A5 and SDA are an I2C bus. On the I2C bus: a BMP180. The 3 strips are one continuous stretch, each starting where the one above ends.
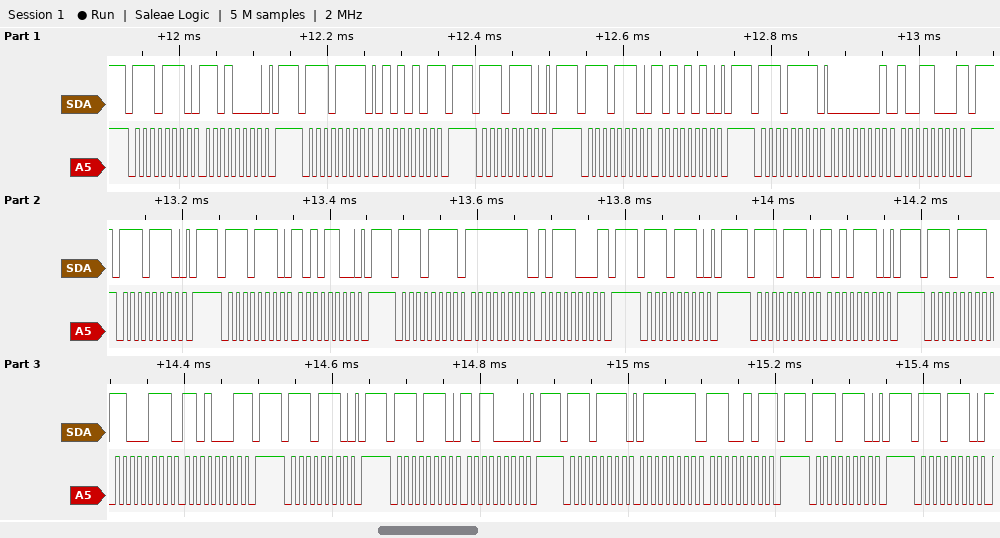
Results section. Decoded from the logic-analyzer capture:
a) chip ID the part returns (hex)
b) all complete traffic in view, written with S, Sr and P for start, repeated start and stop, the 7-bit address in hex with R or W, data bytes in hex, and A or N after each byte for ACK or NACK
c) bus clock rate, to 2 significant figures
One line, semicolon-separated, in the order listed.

0x55; S 77W A D0 A P S 77R A 55 N P S 77W A P S 77W A AA A P S 77R A 01 A 98 N P S 77W A P S 77W A AC A P S 77R A FF A B8 N P S 77W A P S 77W A AE A P S 77R A C7 A D1 N P S 77W A P S 77W A B0 A P S 77R A 7F A E5 N P S 77W A P S 77W A; 100 kHz
